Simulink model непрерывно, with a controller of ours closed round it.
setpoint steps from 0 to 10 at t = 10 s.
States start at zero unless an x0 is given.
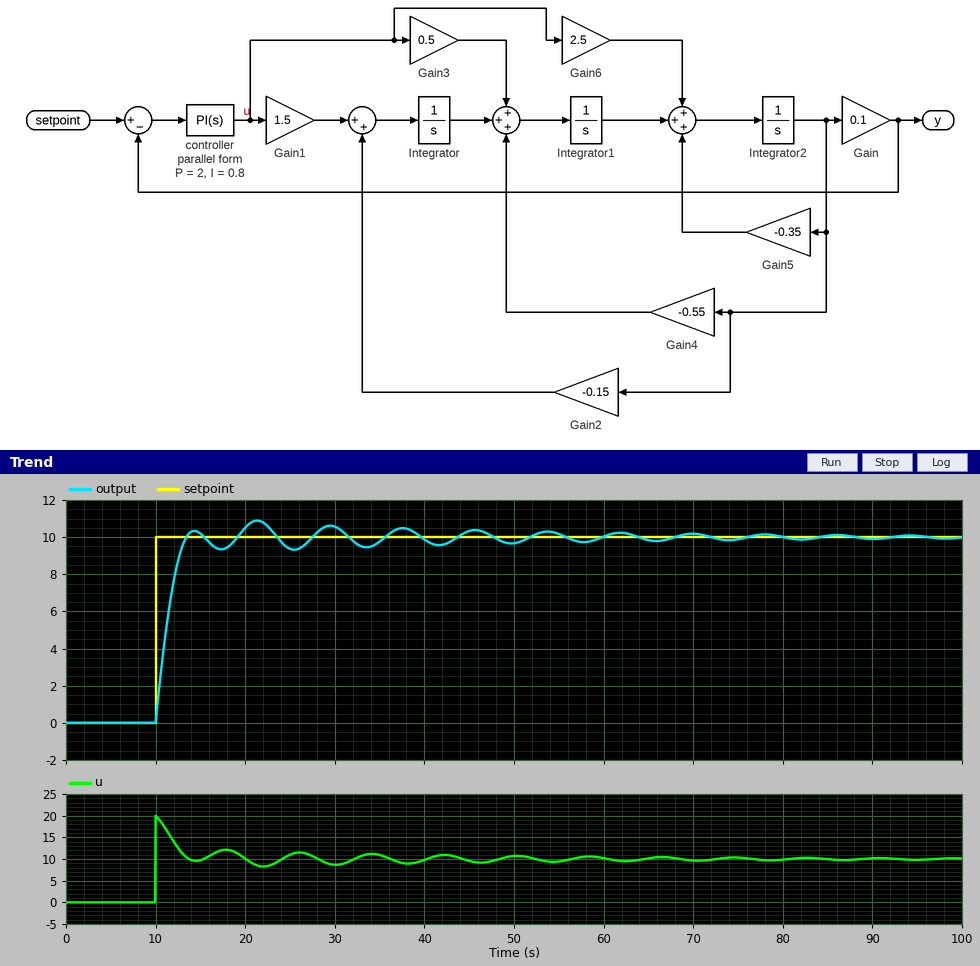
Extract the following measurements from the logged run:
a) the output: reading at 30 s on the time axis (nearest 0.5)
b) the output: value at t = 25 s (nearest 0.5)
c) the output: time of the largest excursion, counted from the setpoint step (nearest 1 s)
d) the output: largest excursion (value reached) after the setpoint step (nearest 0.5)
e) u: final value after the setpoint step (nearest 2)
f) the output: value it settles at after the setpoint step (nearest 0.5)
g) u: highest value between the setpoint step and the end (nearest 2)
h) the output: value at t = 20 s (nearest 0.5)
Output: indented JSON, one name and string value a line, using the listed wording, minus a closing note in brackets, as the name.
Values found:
{
  "the output: reading at 30 s on the time axis": "10.5",
  "the output: value at t = 25 s": "9.5",
  "the output: time of the largest excursion, counted from the setpoint step": "11 s",
  "the output: largest excursion (value reached) after the setpoint step": "11.0",
  "u: final value after the setpoint step": "10",
  "the output: value it settles at after the setpoint step": "10.0",
  "u: highest value between the setpoint step and the end": "20",
  "the output: value at t = 20 s": "10.5"
}
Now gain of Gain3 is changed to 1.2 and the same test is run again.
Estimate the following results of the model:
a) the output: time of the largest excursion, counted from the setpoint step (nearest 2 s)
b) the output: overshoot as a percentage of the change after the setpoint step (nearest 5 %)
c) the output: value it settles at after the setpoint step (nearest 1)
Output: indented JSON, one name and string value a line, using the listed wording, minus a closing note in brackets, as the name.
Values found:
{
  "the output: time of the largest excursion, counted from the setpoint step": "10 s",
  "the output: overshoot as a percentage of the change after the setpoint step": "15 %",
  "the output: value it settles at after the setpoint step": "10"
}
